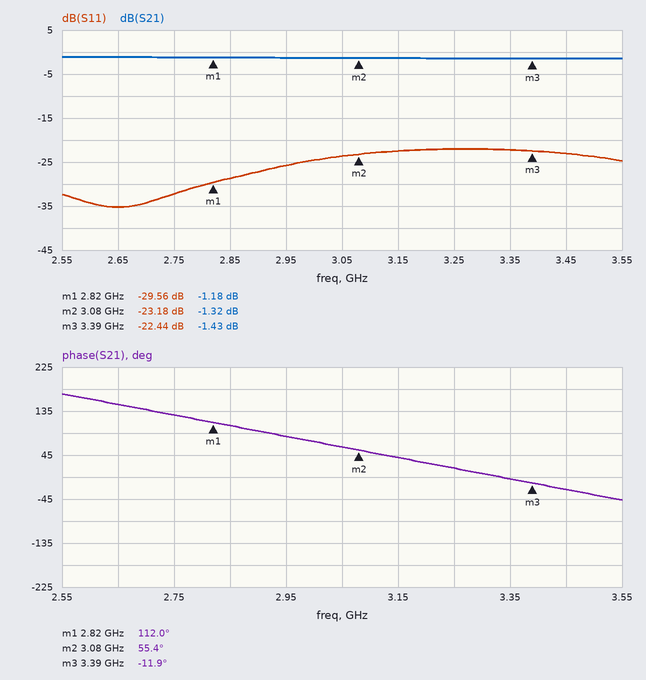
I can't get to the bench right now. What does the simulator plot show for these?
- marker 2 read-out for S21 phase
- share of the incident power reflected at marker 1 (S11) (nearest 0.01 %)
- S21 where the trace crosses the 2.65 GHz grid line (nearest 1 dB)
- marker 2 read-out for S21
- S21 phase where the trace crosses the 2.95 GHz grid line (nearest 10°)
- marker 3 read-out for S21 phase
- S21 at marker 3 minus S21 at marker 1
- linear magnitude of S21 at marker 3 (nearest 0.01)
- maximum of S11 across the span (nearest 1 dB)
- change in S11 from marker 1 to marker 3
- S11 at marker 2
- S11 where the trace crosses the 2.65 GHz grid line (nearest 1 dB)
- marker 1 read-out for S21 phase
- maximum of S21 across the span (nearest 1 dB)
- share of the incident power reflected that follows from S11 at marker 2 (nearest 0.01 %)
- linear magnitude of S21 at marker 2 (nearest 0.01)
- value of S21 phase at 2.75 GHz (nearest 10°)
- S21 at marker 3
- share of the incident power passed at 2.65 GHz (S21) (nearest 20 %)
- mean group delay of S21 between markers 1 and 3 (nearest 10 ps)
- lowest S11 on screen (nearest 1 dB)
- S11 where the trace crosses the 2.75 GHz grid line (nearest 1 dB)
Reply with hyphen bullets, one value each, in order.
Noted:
- 55.4°
- 0.11 %
- -1 dB
- -1.32 dB
- 80°
- -11.9°
- -0.25 dB
- 0.85
- -22 dB
- 7.12 dB
- -23.18 dB
- -35 dB
- 112.0°
- -1 dB
- 0.48 %
- 0.86
- 130°
- -1.43 dB
- 80 %
- 600 ps
- -35 dB
- -32 dB
